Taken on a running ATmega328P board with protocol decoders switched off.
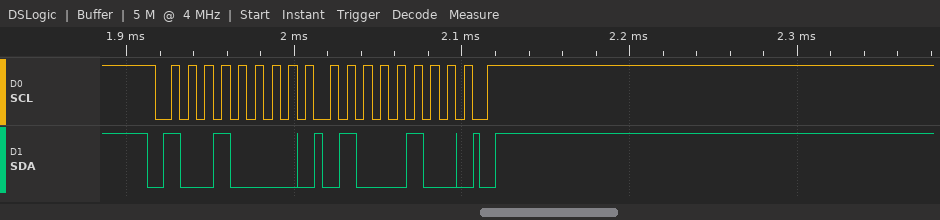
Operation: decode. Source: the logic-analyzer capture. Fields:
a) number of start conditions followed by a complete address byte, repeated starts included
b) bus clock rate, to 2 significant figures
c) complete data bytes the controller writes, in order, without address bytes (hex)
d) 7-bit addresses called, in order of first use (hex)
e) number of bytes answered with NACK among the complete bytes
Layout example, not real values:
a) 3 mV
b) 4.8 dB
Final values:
a) 1
b) 100 kHz
c) 44
d) 0x48
e) 0
